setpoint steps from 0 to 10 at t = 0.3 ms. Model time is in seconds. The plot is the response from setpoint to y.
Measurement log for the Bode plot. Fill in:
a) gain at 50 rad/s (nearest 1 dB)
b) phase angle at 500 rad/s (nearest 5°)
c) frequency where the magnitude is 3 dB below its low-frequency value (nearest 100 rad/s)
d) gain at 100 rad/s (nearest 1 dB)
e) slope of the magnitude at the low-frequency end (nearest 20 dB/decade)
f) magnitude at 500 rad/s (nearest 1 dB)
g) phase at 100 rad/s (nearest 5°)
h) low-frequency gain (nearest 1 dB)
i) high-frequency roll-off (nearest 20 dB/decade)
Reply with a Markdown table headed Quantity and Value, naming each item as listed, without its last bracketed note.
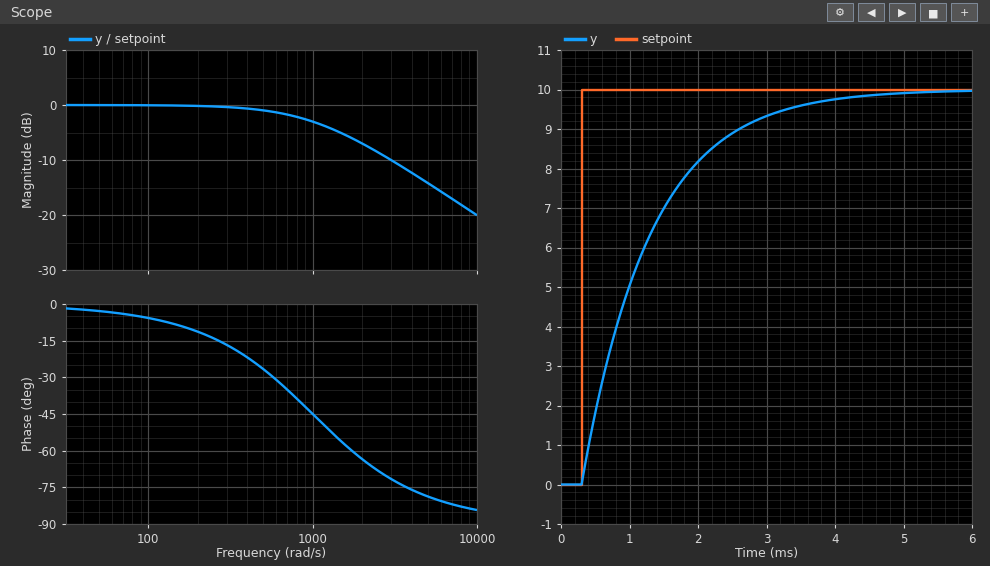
| Quantity | Value |
|---|---|
| gain at 50 rad/s | 0 dB |
| phase angle at 500 rad/s | -25° |
| frequency where the magnitude is 3 dB below its low-frequency value | 1000 rad/s |
| gain at 100 rad/s | 0 dB |
| slope of the magnitude at the low-frequency end | 0 dB/decade |
| magnitude at 500 rad/s | -1 dB |
| phase at 100 rad/s | -5° |
| low-frequency gain | 0 dB |
| high-frequency roll-off | -20 dB/decade |
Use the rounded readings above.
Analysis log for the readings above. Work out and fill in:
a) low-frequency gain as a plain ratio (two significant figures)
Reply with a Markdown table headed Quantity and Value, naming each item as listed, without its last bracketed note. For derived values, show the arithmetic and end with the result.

| Quantity | Value |
|---|---|
| low-frequency gain as a plain ratio | 10^(0 / 20) = 1.0 |
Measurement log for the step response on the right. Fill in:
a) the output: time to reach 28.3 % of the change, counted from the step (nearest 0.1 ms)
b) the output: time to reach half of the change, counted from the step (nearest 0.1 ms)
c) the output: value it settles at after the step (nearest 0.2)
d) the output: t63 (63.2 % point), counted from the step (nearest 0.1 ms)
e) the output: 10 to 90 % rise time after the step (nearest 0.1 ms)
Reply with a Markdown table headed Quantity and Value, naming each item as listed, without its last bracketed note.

| Quantity | Value |
|---|---|
| the output: time to reach 28.3 % of the change, counted from the step | 0.3 ms |
| the output: time to reach half of the change, counted from the step | 0.7 ms |
| the output: value it settles at after the step | 10.0 |
| the output: t63 (63.2 % point), counted from the step | 1.0 ms |
| the output: 10 to 90 % rise time after the step | 2.2 ms |
